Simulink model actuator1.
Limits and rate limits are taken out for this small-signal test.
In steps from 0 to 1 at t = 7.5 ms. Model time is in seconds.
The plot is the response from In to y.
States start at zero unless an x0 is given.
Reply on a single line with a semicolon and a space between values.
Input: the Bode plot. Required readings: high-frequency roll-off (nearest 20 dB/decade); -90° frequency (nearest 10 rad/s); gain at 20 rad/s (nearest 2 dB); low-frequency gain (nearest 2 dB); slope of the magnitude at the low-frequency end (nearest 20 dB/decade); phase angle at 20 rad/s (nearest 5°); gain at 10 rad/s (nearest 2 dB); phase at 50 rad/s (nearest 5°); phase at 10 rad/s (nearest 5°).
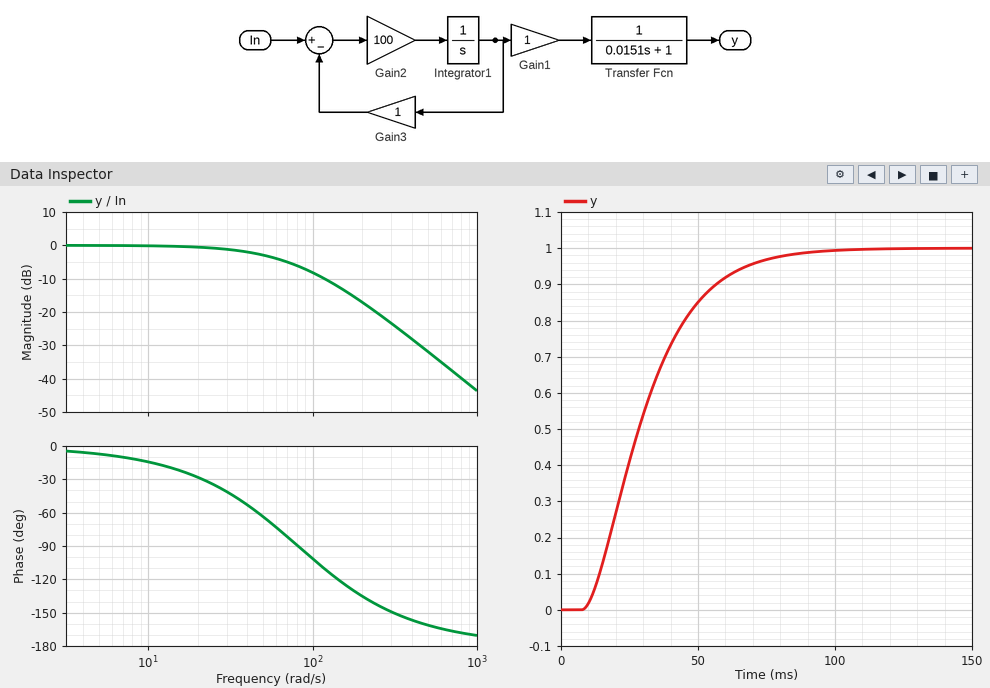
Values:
-40 dB/decade; 80 rad/s; 0 dB; 0 dB; 0 dB/decade; -30°; 0 dB; -65°; -15°
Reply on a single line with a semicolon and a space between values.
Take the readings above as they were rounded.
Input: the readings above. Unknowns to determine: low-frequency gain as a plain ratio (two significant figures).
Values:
1.0
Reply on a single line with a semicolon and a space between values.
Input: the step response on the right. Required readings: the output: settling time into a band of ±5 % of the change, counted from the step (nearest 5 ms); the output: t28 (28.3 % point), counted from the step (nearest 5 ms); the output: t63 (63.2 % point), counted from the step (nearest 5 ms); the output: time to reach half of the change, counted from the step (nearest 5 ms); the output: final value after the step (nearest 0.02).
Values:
60 ms; 15 ms; 25 ms; 20 ms; 1.00
